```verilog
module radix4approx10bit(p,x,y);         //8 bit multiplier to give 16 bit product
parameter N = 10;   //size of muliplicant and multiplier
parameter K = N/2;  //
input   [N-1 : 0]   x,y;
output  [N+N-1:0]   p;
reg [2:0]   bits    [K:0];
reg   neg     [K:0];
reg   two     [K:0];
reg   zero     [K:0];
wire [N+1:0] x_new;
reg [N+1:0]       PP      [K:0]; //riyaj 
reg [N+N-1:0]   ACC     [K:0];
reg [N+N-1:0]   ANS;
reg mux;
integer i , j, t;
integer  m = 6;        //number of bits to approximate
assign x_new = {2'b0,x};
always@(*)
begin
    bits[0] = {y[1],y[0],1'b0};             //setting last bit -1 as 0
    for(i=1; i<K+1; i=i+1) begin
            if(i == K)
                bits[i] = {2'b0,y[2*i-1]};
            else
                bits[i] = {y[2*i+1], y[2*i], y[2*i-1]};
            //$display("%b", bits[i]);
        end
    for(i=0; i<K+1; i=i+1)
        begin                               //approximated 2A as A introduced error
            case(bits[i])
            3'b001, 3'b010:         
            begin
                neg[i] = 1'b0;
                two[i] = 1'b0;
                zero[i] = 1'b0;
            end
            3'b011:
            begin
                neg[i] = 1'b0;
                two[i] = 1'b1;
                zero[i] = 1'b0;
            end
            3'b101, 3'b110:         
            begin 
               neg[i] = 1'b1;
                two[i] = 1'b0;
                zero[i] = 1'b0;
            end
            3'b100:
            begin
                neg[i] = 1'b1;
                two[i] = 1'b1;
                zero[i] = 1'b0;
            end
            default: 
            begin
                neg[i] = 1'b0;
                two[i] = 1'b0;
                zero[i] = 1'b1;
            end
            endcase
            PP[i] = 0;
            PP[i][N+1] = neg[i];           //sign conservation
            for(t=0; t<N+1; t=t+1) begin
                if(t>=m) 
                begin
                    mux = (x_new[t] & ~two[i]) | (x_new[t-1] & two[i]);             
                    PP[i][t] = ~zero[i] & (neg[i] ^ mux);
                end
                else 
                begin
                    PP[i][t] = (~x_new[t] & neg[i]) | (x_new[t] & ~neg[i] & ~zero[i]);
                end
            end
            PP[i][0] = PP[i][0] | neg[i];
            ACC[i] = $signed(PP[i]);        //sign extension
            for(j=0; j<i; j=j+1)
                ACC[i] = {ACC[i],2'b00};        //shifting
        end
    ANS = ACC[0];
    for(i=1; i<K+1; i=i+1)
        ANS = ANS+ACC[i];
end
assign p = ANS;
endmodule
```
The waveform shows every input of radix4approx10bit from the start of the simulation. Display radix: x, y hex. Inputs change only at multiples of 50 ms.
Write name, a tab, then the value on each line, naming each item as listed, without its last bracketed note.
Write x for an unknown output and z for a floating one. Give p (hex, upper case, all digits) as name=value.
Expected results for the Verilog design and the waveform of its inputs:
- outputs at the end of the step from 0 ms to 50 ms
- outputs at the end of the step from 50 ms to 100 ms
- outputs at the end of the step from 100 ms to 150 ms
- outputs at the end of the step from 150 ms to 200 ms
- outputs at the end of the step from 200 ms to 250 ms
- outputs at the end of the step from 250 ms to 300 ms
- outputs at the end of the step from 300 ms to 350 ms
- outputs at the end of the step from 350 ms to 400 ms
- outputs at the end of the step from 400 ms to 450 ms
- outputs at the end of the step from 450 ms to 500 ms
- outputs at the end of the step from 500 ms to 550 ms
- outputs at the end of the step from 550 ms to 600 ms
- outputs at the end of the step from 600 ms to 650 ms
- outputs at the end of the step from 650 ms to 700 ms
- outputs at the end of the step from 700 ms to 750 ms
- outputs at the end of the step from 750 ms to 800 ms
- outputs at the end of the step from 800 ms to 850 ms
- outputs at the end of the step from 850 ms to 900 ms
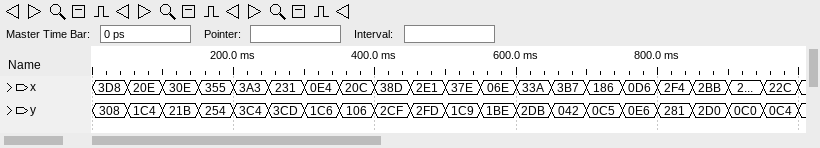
outputs at the end of the step from 0 ms to 50 ms	p=BA61C
outputs at the end of the step from 50 ms to 100 ms	p=39278
outputs at the end of the step from 100 ms to 150 ms	p=67A95
outputs at the end of the step from 150 ms to 200 ms	p=7D6E4
outputs at the end of the step from 200 ms to 250 ms	p=DB1CC
outputs at the end of the step from 250 ms to 300 ms	p=8543D
outputs at the end of the step from 300 ms to 350 ms	p=1B06B
outputs at the end of the step from 350 ms to 400 ms	p=21823
outputs at the end of the step from 400 ms to 450 ms	p=9F903
outputs at the end of the step from 450 ms to 500 ms	p=89A5D
outputs at the end of the step from 500 ms to 550 ms	p=63DA2
outputs at the end of the step from 550 ms to 600 ms	p=0D151
outputs at the end of the step from 600 ms to 650 ms	p=935B9
outputs at the end of the step from 650 ms to 700 ms	p=0F525
outputs at the end of the step from 700 ms to 750 ms	p=12BDE
outputs at the end of the step from 750 ms to 800 ms	p=0C151
outputs at the end of the step from 800 ms to 850 ms	p=760B4
outputs at the end of the step from 850 ms to 900 ms	p=7ADF0
